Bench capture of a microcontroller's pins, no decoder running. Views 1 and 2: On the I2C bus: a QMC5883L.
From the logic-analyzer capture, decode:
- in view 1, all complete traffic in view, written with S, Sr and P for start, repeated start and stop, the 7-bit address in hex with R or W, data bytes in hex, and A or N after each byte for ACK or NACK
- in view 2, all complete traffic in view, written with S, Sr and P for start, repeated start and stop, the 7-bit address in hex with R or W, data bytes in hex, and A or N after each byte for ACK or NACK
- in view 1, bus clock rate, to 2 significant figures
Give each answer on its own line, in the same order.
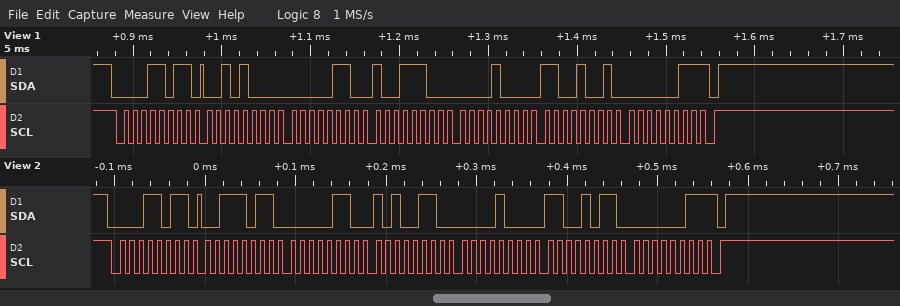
S 0DR A 28 A 06 A 9C A 08 A C9 A 03 N P
S 0DR A 3B A 06 A A6 A 08 A CB A 03 N P
100 kHz
